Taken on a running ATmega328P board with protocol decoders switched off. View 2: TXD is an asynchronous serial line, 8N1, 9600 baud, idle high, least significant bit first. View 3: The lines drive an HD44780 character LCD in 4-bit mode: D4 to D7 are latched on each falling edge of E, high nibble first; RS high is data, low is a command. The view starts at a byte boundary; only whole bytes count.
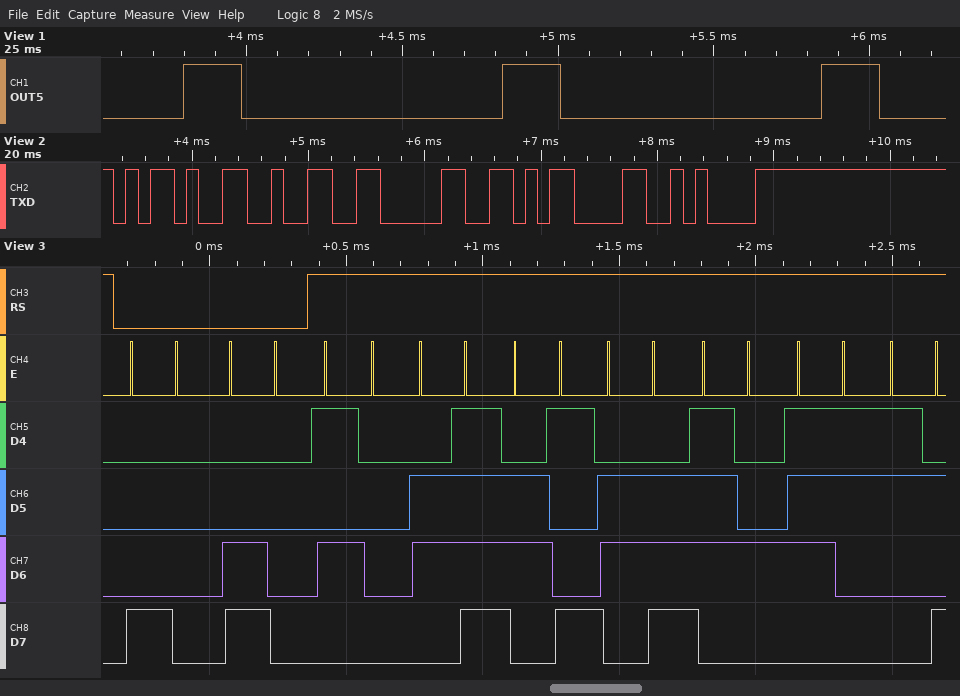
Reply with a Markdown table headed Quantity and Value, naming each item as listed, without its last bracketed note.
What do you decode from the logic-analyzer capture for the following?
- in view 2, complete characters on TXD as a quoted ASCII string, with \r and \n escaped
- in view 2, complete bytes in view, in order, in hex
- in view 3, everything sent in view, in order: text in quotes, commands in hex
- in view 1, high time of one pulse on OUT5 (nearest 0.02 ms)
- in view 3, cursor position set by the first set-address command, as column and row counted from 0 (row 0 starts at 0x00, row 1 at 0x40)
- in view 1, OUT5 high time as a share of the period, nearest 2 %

| Quantity | Value |
|---|---|
| in view 2, complete characters on TXD as a quoted ASCII string, with \r and \n escaped | "-20\r\n" |
| in view 2, complete bytes in view, in order, in hex | 0x2D 0x32 0x30 0x0D 0x0A |
| in view 3, everything sent in view, in order: text in quotes, commands in hex | 0x80 0xC0 "Points:" |
| in view 1, high time of one pulse on OUT5 | 0.18 ms |
| in view 3, cursor position set by the first set-address command, as column and row counted from 0 | column 0, row 0 |
| in view 1, OUT5 high time as a share of the period, nearest 2 % | 18 % |
